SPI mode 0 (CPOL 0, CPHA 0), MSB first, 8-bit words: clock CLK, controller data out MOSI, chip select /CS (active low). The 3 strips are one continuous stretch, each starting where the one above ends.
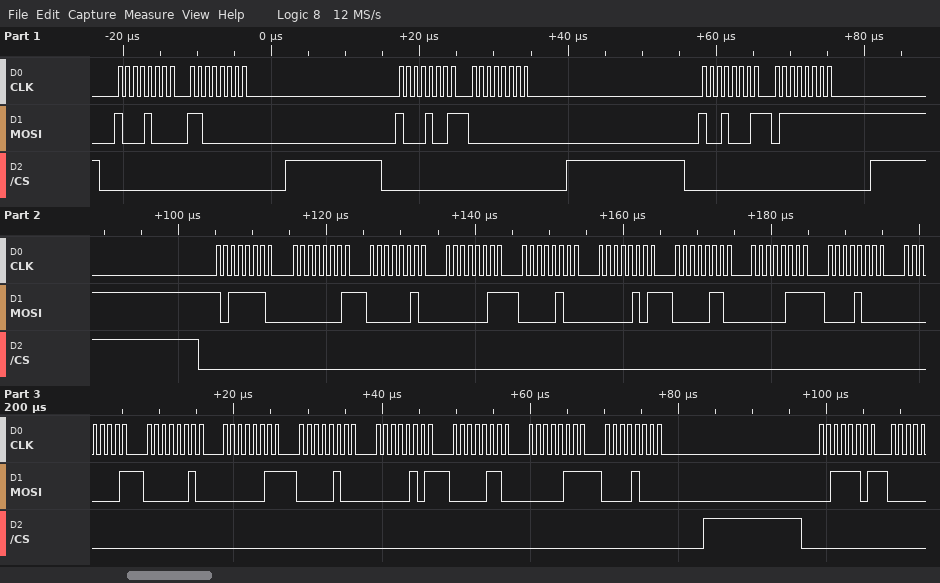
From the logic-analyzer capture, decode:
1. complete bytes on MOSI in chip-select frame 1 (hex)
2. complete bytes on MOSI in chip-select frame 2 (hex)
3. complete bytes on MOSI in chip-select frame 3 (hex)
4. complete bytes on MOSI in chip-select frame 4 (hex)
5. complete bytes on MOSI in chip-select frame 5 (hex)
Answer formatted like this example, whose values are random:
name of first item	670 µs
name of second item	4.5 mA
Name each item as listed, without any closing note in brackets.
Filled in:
complete bytes on MOSI in chip-select frame 1	88 C0
complete bytes on MOSI in chip-select frame 2	89 00
complete bytes on MOSI in chip-select frame 3	91 7F
complete bytes on MOSI in chip-select frame 4	BE 01 02 03 04 05 06 07 08 01 02 03 04 05 06 07 08
complete bytes on MOSI in chip-select frame 5	3D
